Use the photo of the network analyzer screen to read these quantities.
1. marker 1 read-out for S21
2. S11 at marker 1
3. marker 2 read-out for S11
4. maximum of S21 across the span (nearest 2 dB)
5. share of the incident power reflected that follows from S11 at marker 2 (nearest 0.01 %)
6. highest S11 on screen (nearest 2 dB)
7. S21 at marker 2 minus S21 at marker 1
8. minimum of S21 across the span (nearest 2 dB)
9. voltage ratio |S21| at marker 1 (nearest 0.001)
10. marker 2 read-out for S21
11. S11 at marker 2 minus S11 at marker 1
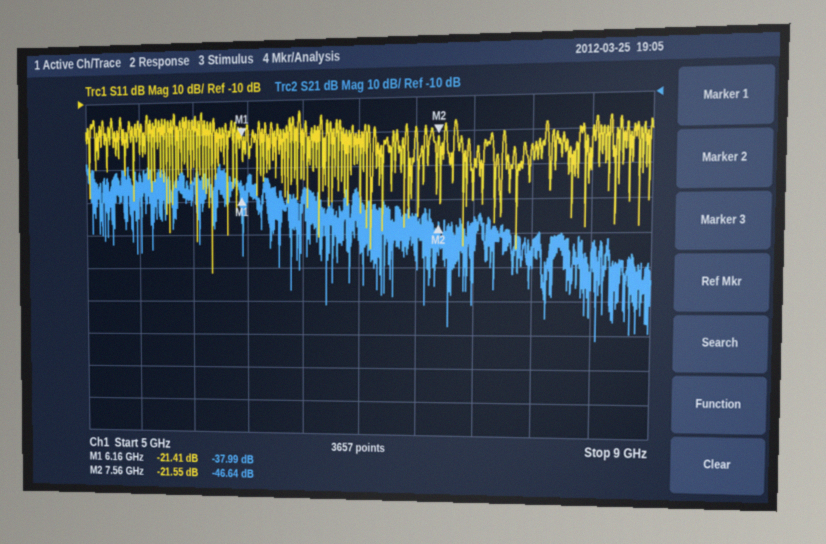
-37.99 dB
-21.41 dB
-21.55 dB
-28 dB
0.70 %
-14 dB
-8.65 dB
-82 dB
0.013
-46.64 dB
-0.14 dB
